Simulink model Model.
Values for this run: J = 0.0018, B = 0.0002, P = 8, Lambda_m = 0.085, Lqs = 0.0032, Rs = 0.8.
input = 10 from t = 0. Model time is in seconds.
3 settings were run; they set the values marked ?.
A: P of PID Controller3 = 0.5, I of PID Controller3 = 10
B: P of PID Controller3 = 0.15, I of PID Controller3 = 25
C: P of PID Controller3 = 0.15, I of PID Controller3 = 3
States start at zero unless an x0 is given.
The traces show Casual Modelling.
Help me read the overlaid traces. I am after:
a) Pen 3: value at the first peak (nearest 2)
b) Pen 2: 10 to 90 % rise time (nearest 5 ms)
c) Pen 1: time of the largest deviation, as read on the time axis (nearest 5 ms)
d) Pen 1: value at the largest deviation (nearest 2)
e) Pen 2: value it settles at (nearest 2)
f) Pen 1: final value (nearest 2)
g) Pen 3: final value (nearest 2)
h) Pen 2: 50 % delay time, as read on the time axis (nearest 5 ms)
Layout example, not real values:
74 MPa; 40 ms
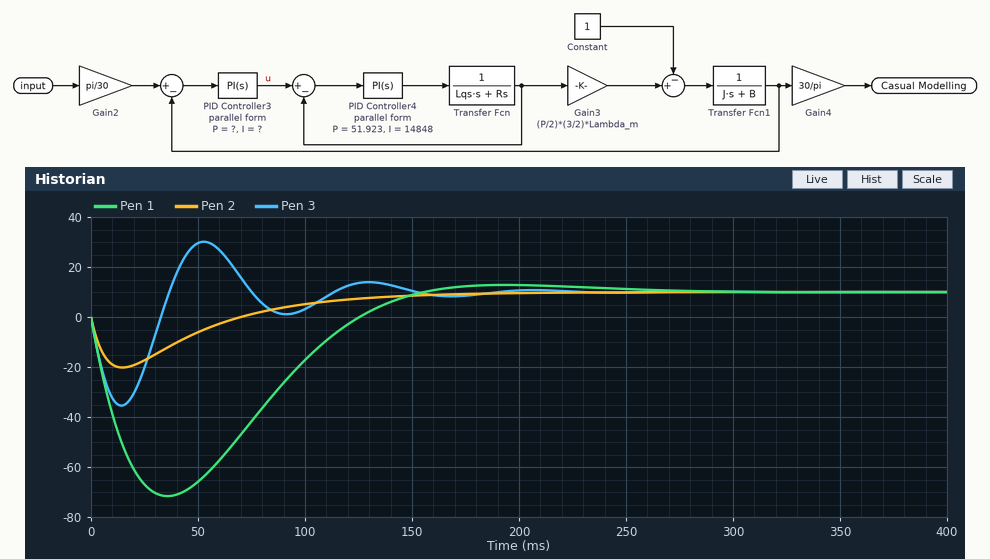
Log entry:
30; 90 ms; 35 ms; -72; 10; 10; 10; 100 ms
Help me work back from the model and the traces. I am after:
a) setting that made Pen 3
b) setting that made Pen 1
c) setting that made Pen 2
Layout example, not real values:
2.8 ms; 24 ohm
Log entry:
B; C; A
